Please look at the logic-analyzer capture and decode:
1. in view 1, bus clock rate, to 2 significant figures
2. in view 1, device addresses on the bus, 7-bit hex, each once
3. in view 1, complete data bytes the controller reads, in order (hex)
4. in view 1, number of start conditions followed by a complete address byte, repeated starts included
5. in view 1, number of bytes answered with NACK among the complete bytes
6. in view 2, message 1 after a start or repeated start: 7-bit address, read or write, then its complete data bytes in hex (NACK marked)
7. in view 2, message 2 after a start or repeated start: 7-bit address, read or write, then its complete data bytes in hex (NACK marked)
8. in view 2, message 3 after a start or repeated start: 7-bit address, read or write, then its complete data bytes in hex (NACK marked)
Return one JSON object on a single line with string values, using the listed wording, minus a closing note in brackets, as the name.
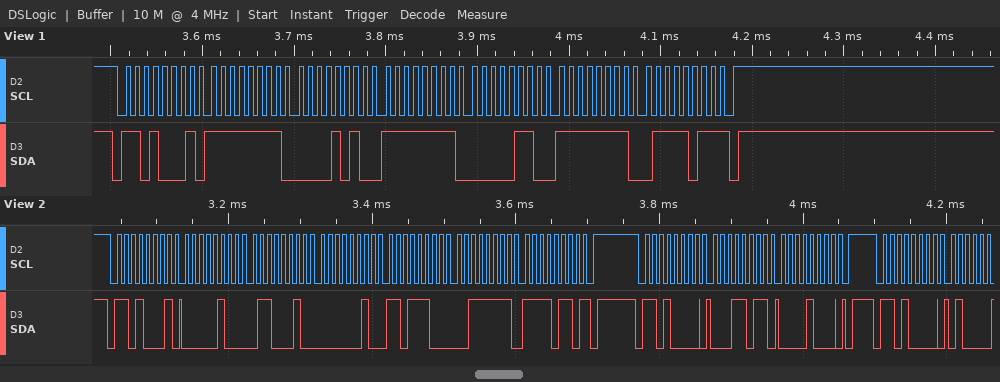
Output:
{"in view 1, bus clock rate, to 2 significant figures": "100 kHz", "in view 1, device addresses on the bus, 7-bit hex, each once": "0x68", "in view 1, complete data bytes the controller reads, in order": "FF 0A FF 06 FF 7B", "in view 1, number of start conditions followed by a complete address byte, repeated starts included": "1", "in view 1, number of bytes answered with NACK among the complete bytes": "1", "in view 2, message 1 after a start or repeated start: 7-bit address, read or write, then its complete data bytes in hex": "0x68 read: 04 62 02 DC 3F F6 NACK", "in view 2, message 2 after a start or repeated start: 7-bit address, read or write, then its complete data bytes in hex": "0x68 write: 1B 08", "in view 2, message 3 after a start or repeated start: 7-bit address, read or write, then its complete data bytes in hex": "0x68 write"}
